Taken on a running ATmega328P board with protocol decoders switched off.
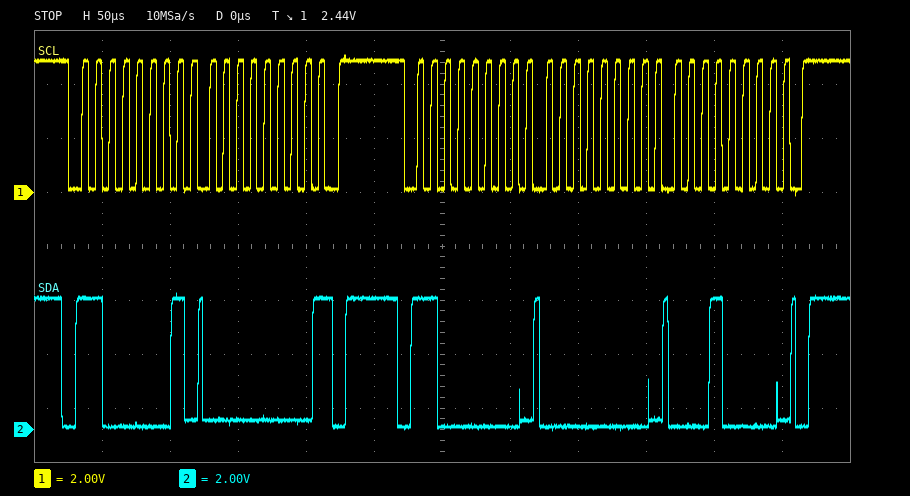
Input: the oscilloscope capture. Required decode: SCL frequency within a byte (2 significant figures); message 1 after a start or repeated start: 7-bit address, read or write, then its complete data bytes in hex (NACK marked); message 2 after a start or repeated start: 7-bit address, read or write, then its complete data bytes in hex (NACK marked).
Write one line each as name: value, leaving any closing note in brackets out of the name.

SCL frequency within a byte: 100 kHz
message 1 after a start or repeated start: 7-bit address, read or write, then its complete data bytes in hex: 0x60 read: 00 NACK
message 2 after a start or repeated start: 7-bit address, read or write, then its complete data bytes in hex: 0x60 write: 00 10
